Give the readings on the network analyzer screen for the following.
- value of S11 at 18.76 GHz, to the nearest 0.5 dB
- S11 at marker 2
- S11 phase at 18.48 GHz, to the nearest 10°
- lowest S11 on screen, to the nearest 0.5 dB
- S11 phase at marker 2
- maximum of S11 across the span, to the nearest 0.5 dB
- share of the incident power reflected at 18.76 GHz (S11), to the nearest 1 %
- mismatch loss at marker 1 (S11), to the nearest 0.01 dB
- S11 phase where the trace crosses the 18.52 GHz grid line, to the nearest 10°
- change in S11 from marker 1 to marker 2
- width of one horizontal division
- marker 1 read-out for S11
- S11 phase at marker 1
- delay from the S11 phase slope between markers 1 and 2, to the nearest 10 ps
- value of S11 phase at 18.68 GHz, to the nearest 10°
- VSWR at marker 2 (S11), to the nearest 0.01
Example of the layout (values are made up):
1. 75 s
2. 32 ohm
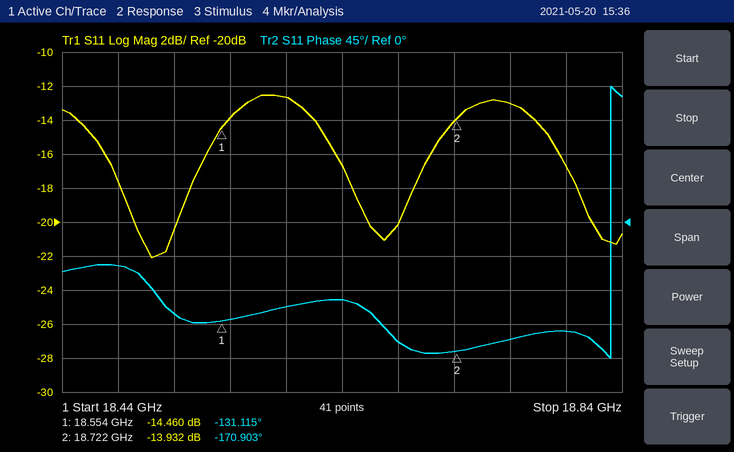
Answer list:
1. -13.0 dB
2. -13.932 dB
3. -60°
4. -22.0 dB
5. -170.903°
6. -12.5 dB
7. 5 %
8. 0.16 dB
9. -120°
10. 0.528 dB
11. 40 MHz
12. -14.460 dB
13. -131.115°
14. 660 ps
15. -160°
16. 1.50
